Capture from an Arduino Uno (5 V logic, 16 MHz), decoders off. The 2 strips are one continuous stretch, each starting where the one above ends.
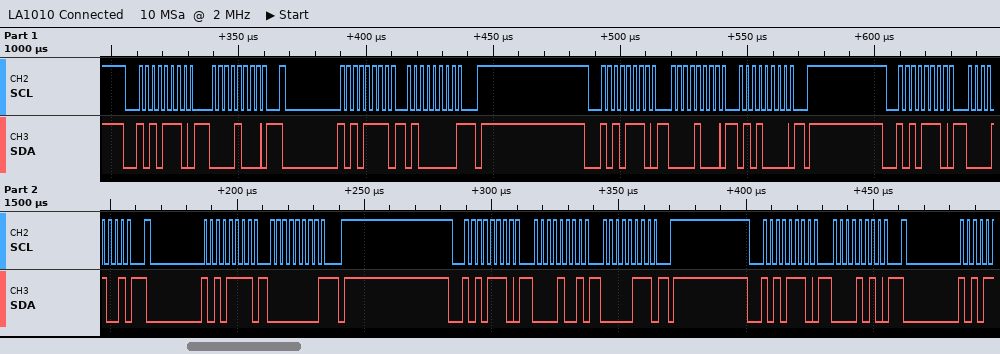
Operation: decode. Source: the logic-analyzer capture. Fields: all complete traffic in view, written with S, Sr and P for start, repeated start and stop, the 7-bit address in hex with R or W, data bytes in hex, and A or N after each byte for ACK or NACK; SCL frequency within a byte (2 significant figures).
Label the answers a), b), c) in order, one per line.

a) S 57W A 08 A Sr 57R A 40 N P S 57W A 08 A 50 A P S 57W A 09 A Sr 57R A 00 N P S 57W A 09 A 07 A P S 57W A 0A A
b) 400 kHz
